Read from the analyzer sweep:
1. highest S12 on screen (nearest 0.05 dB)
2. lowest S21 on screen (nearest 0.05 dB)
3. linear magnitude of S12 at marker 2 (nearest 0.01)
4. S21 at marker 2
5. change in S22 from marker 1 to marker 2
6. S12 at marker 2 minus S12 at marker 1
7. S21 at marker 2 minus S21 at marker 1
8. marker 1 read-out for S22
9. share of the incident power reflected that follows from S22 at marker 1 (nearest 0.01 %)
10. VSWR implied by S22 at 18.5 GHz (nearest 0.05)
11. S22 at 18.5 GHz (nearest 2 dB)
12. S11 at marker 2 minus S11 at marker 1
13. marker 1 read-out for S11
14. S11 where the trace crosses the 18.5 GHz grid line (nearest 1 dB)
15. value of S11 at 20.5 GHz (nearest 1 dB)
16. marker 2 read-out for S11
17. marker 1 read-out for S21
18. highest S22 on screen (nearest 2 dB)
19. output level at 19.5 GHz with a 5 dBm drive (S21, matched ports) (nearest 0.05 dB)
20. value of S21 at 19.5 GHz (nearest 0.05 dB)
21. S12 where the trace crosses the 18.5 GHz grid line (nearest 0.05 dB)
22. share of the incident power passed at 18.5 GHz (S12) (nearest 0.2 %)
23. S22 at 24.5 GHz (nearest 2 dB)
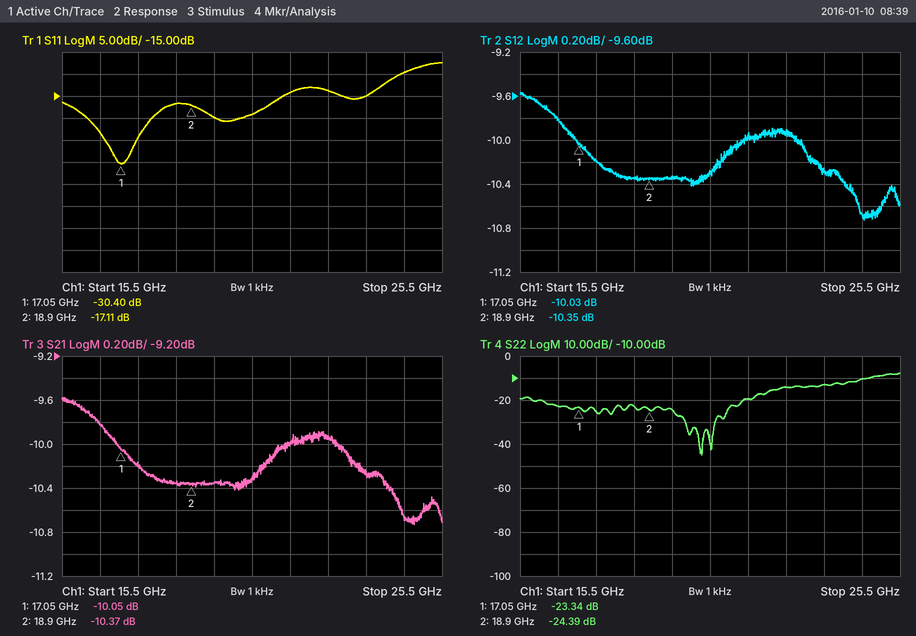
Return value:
-9.55 dB
-10.75 dB
0.30
-10.37 dB
-1.05 dB
-0.32 dB
-0.32 dB
-23.34 dB
0.46 %
1.15
-22 dB
13.29 dB
-30.40 dB
-17 dB
-19 dB
-17.11 dB
-10.05 dB
-8 dB
-5.35 dBm
-10.35 dB
-10.35 dB
9.2 %
-10 dB
